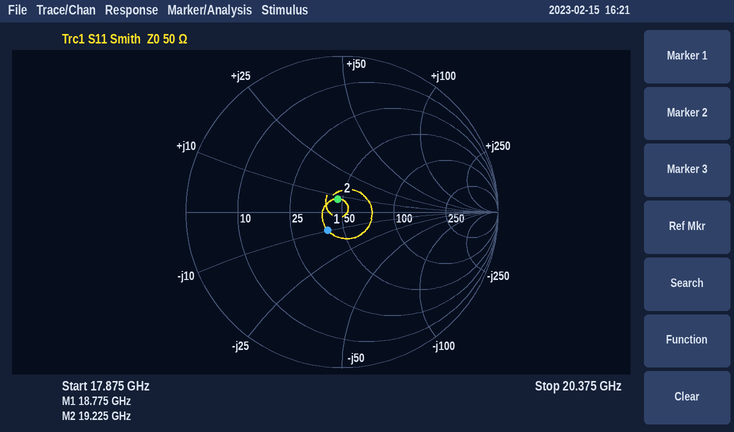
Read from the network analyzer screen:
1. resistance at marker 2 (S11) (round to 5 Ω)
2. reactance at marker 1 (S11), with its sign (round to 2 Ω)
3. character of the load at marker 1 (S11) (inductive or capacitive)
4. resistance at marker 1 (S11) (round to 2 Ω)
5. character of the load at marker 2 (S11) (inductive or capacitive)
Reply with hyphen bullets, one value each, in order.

- 45 Ω
- -10 Ω
- capacitive
- 40 Ω
- inductive
